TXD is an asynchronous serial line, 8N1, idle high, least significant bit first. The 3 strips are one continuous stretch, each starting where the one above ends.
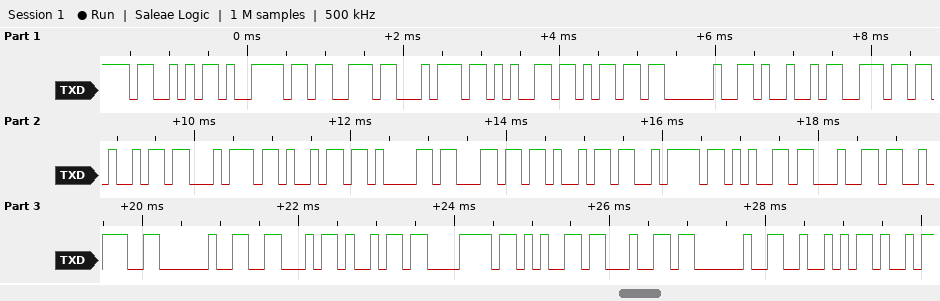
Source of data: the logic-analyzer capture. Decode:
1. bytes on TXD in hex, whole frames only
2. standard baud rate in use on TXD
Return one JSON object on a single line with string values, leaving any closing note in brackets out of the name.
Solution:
{"bytes on TXD in hex, whole frames only": "0x53 0x79 0x73 0x74 0x65 0x6D 0x20 0x49 0x6E 0x69 0x74 0x69 0x61 0x6C 0x69 0x7A 0x65 0x64 0x3A 0x20 0x46 0x69 0x78 0x65 0x64 0x20 0x52", "standard baud rate in use on TXD": "9600 baud"}
